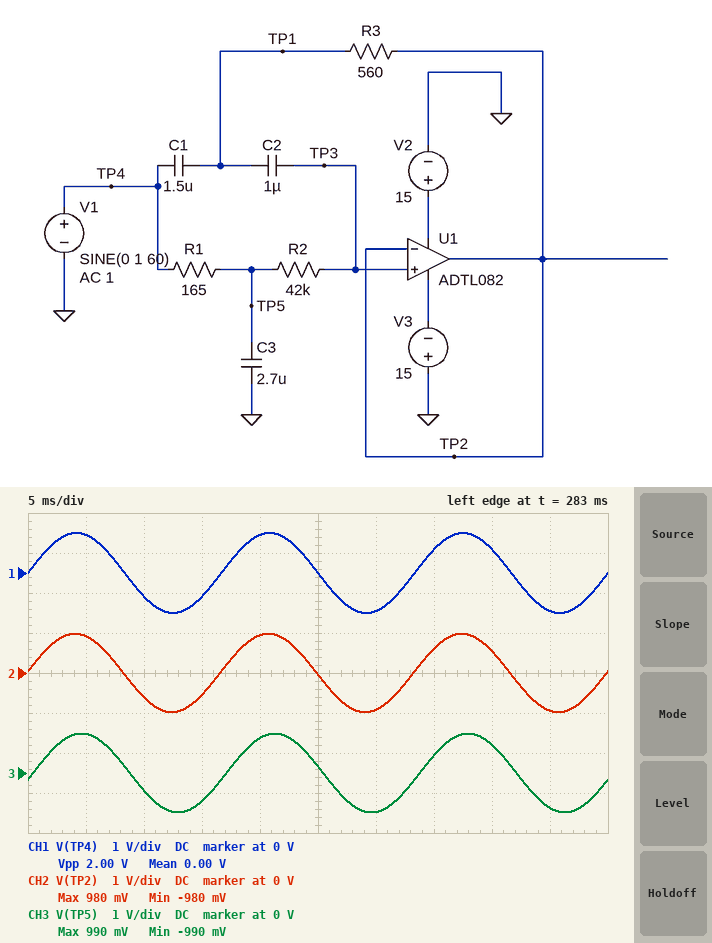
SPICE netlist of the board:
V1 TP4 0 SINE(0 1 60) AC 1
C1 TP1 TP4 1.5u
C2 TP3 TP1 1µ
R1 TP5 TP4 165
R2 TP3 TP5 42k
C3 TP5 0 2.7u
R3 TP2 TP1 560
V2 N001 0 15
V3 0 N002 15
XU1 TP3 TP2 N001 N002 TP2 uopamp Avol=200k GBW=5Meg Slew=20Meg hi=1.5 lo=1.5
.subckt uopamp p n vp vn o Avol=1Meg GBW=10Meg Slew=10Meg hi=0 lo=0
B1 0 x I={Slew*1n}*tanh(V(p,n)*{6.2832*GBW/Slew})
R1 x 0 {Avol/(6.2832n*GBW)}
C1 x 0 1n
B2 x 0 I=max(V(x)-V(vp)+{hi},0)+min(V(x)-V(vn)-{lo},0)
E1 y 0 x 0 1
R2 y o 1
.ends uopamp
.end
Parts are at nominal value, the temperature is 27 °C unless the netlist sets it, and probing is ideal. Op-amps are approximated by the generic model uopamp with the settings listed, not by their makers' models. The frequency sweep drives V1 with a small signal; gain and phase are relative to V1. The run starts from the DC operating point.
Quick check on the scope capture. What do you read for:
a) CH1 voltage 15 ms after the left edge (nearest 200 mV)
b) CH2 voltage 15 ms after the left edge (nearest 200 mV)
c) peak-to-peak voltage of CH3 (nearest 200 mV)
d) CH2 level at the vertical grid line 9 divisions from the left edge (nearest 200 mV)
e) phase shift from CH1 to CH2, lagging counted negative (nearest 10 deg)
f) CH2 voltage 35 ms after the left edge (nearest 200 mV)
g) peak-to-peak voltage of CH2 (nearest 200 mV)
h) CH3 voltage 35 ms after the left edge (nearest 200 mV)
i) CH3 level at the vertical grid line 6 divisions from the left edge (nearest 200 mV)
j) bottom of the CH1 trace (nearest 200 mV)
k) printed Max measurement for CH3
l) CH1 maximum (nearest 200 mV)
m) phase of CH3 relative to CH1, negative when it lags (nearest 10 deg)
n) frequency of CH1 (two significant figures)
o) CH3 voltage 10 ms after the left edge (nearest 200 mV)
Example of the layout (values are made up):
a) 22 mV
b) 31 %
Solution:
a) -600 mV
b) -600 mV
c) 2.0 V
d) -1.0 V
e) 0 deg
f) 600 mV
g) 2.0 V
h) 400 mV
i) -1.0 V
j) -1.0 V
k) 990 mV
l) 1.0 V
m) -10 deg
n) 60 Hz
o) -400 mV
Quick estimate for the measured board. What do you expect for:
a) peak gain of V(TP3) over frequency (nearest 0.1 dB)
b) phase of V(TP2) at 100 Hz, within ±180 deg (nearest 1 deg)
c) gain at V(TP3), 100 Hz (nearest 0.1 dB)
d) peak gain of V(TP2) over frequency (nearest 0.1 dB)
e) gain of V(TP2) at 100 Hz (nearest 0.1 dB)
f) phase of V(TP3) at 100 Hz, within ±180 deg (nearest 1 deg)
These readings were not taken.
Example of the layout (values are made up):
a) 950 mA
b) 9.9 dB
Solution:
a) 0 dB
b) 1 deg
c) -0.1 dB
d) 0 dB
e) -0.1 dB
f) 1 deg
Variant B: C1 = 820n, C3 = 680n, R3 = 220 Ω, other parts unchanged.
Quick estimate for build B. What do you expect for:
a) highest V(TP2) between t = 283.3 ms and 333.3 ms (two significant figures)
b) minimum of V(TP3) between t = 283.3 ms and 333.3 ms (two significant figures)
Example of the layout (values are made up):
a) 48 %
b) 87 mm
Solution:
a) 770 mV
b) -770 mV
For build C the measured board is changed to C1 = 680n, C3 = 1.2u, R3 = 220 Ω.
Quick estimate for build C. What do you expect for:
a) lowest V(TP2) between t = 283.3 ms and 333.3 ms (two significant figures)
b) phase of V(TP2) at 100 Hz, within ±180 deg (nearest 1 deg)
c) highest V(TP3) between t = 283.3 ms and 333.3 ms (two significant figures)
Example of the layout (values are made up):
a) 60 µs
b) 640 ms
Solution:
a) -730 mV
b) 5 deg
c) 730 mV
